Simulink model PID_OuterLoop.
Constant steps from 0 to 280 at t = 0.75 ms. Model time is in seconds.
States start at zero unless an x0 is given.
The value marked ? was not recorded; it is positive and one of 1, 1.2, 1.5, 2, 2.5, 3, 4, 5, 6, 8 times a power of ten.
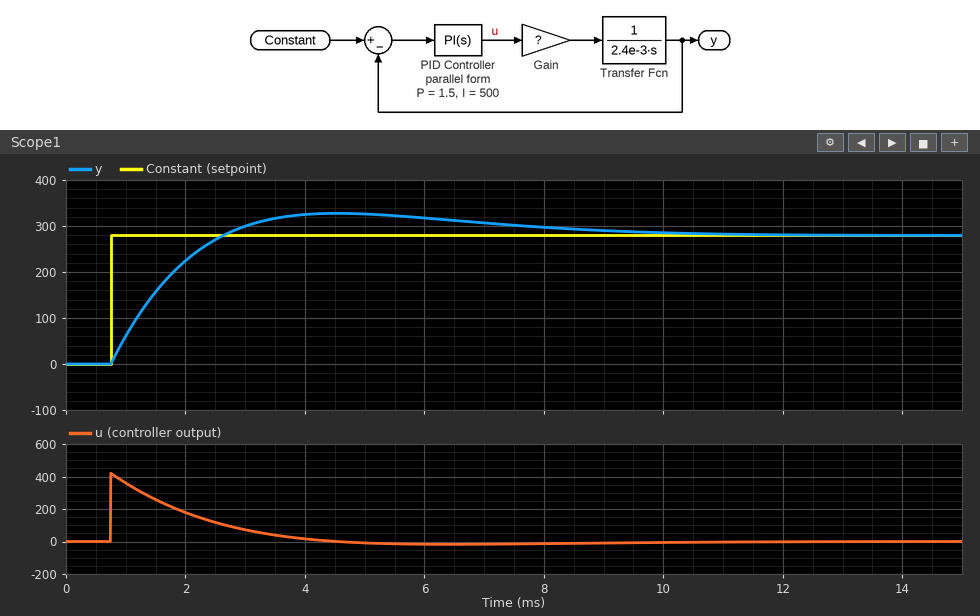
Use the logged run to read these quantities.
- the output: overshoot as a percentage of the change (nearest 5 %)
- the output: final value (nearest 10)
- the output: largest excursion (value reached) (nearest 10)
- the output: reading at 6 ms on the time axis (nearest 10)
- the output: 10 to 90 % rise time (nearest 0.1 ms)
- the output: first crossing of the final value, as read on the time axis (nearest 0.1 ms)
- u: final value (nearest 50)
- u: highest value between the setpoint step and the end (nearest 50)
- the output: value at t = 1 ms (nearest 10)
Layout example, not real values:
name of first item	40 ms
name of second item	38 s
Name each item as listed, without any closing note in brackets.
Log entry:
the output: overshoot as a percentage of the change	15 %
the output: final value	280
the output: largest excursion (value reached)	330
the output: reading at 6 ms on the time axis	320
the output: 10 to 90 % rise time	1.4 ms
the output: first crossing of the final value, as read on the time axis	2.6 ms
u: final value	0
u: highest value between the setpoint step and the end	400
the output: value at t = 1 ms	60
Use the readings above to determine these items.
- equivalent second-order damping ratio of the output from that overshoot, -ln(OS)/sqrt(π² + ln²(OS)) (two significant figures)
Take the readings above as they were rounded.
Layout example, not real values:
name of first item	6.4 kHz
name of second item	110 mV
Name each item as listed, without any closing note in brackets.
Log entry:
equivalent second-order damping ratio of the output from that overshoot, -ln(OS)/sqrt(π² + ln²(OS))	0.52
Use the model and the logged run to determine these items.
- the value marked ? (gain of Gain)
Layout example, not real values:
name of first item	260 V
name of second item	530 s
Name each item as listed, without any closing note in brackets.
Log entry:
the value marked ?	1.5
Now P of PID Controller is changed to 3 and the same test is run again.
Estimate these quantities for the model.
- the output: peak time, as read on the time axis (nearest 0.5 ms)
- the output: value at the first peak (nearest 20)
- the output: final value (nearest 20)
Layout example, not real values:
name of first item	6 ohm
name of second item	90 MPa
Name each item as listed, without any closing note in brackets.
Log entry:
the output: peak time, as read on the time axis	3.5 ms
the output: value at the first peak	300
the output: final value	280
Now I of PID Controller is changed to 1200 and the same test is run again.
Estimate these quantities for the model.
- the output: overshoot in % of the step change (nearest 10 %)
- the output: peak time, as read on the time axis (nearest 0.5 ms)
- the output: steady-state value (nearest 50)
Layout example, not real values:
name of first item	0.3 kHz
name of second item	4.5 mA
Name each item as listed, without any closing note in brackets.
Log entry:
the output: overshoot in % of the step change	30 %
the output: peak time, as read on the time axis	3.5 ms
the output: steady-state value	300
